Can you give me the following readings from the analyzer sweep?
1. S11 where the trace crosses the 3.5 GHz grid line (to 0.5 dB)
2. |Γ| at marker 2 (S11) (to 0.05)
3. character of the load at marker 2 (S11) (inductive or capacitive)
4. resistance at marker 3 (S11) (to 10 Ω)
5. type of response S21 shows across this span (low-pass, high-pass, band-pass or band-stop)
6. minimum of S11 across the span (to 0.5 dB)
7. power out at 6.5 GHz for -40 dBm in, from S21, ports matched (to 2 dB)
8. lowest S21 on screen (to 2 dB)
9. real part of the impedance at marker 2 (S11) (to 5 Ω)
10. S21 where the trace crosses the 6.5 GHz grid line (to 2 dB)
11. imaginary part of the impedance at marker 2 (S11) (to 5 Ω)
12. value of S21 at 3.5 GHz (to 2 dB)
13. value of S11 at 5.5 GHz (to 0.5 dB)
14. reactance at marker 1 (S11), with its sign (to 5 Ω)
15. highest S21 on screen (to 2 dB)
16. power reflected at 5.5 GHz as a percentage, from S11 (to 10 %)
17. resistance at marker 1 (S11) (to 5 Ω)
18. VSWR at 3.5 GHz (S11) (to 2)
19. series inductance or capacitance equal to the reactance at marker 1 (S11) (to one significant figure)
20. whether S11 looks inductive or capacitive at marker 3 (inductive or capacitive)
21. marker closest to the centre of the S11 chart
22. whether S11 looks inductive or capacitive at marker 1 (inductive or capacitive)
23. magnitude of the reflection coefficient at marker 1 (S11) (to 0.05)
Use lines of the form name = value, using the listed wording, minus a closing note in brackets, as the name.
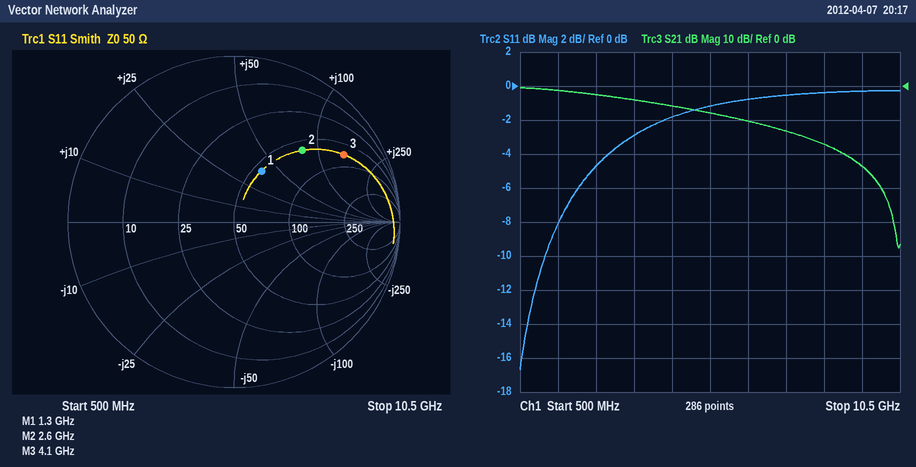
S11 where the trace crosses the 3.5 GHz grid line = -3.0 dB
|Γ| at marker 2 (S11) = 0.60
character of the load at marker 2 (S11) = inductive
resistance at marker 3 (S11) = 70 Ω
type of response S21 shows across this span = low-pass
minimum of S11 across the span = -16.5 dB
power out at 6.5 GHz for -40 dBm in, from S21, ports matched = -50 dBm
lowest S21 on screen = -48 dB
real part of the impedance at marker 2 (S11) = 60 Ω
S21 where the trace crosses the 6.5 GHz grid line = -10 dB
imaginary part of the impedance at marker 2 (S11) = +80 Ω
value of S21 at 3.5 GHz = -4 dB
value of S11 at 5.5 GHz = -1.0 dB
reactance at marker 1 (S11), with its sign = +40 Ω
highest S21 on screen = 0 dB
power reflected at 5.5 GHz as a percentage, from S11 = 80 %
resistance at marker 1 (S11) = 55 Ω
VSWR at 3.5 GHz (S11) = 6
series inductance or capacitance equal to the reactance at marker 1 (S11) = 5 nH
whether S11 looks inductive or capacitive at marker 3 = inductive
marker closest to the centre of the S11 chart = marker 1
whether S11 looks inductive or capacitive at marker 1 = inductive
magnitude of the reflection coefficient at marker 1 (S11) = 0.35
